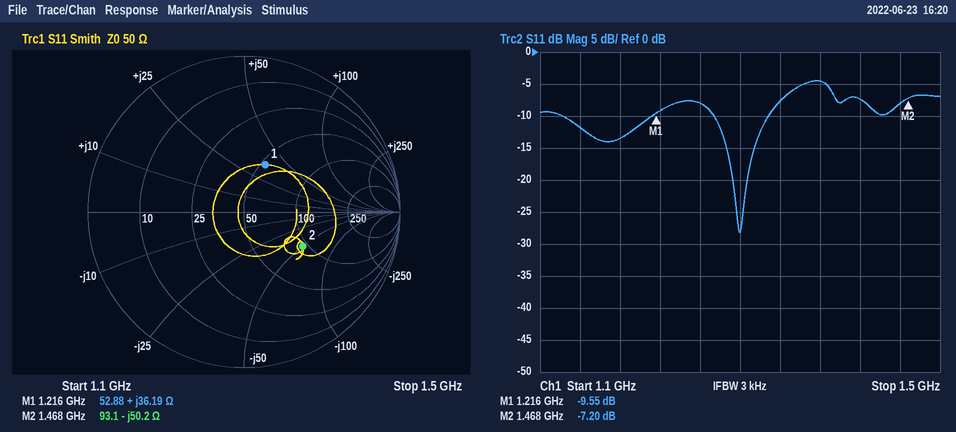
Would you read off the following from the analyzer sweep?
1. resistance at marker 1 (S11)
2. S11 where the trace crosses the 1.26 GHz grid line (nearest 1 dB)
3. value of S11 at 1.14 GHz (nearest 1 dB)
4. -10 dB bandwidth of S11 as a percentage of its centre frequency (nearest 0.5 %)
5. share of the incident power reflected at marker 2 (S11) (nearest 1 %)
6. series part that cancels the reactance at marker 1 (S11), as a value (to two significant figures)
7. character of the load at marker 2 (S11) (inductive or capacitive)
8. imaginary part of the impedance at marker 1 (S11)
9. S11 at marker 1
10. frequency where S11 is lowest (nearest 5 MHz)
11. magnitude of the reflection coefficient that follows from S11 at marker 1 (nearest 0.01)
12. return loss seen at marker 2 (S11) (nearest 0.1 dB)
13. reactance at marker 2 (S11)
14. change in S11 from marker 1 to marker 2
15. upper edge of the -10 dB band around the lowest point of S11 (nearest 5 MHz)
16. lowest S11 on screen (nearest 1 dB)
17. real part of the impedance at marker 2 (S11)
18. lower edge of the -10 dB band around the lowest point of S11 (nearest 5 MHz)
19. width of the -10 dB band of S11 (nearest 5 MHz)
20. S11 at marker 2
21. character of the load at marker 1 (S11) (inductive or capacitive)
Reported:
52.88 Ω
-8 dB
-12 dB
4.0 %
19 %
3.6 pF
capacitive
+36.19 Ω
-9.55 dB
1.300 GHz
0.33
7.2 dB
-50.2 Ω
2.35 dB
1.330 GHz
-28 dB
93.1 Ω
1.275 GHz
55 MHz
-7.20 dB
inductive
